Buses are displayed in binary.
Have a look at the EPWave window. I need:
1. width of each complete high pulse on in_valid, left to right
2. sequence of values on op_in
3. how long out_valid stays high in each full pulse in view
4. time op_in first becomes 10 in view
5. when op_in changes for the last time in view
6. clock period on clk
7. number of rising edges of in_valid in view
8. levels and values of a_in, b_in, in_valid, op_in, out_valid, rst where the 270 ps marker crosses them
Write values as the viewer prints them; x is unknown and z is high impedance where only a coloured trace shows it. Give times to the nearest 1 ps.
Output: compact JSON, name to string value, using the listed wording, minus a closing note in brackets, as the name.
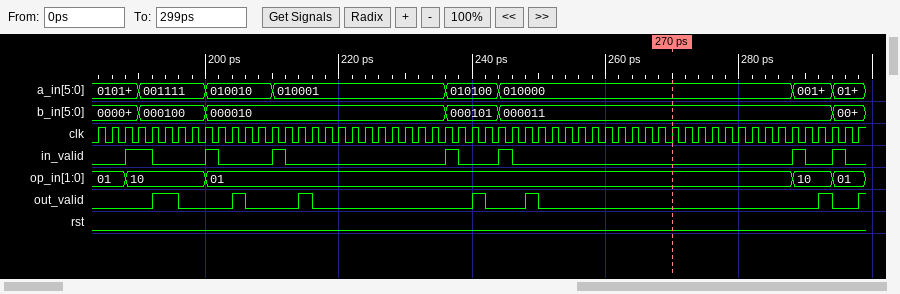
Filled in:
{"width of each complete high pulse on in_valid, left to right": "4 ps, 2 ps, 2 ps, 2 ps, 2 ps, 2 ps, 2 ps", "sequence of values on op_in": "01, 10, 01, 10, 01", "how long out_valid stays high in each full pulse in view": "4 ps, 2 ps, 2 ps, 2 ps, 2 ps, 2 ps", "time op_in first becomes 10 in view": "188 ps", "when op_in changes for the last time in view": "294 ps", "clock period on clk": "2 ps", "number of rising edges of in_valid in view": "7", "levels and values of a_in, b_in, in_valid, op_in, out_valid, rst where the 270 ps marker crosses them": "a_in=010000, b_in=000011, in_valid=0, op_in=01, out_valid=0, rst=0"}
